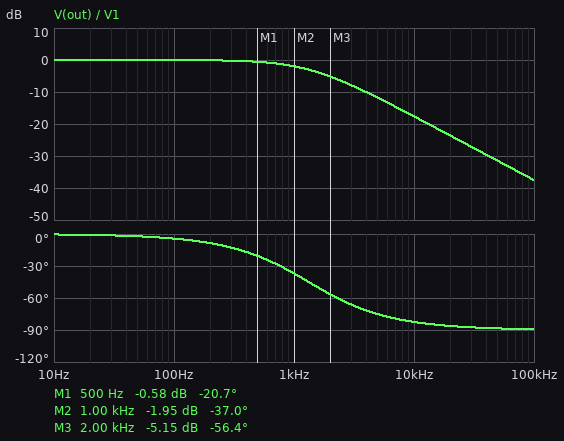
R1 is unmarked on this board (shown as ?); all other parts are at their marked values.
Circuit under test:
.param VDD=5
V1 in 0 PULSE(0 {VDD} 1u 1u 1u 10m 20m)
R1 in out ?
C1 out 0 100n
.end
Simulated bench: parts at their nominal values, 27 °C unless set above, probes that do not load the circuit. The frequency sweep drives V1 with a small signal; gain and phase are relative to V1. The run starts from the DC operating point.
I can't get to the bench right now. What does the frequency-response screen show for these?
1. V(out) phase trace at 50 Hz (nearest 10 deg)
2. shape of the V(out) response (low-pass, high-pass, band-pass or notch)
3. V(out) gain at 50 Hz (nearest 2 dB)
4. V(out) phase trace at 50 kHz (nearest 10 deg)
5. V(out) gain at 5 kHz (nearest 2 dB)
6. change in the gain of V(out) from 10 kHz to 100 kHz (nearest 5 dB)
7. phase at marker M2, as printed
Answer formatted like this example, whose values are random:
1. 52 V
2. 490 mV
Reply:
1. 0 deg
2. low-pass
3. 0 dB
4. -90 deg
5. -12 dB
6. -20 dB
7. -37.0 deg
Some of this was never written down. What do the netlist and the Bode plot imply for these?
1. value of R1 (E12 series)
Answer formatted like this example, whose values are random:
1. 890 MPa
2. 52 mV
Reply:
1. 1.2 kΩ
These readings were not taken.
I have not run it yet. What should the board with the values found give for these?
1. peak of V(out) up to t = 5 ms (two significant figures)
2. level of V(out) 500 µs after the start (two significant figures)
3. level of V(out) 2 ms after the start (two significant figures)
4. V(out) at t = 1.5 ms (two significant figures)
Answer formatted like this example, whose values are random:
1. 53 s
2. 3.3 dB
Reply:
1. 5.0 V
2. 4.9 V
3. 5.0 V
4. 5.0 V
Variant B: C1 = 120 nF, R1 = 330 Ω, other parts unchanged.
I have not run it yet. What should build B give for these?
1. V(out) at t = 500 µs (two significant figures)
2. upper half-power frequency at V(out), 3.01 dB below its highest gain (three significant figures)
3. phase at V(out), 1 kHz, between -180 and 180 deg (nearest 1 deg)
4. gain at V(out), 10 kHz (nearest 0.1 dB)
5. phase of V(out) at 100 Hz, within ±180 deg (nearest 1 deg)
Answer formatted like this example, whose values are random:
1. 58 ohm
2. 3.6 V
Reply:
1. 5.0 V
2. 4.02 kHz
3. -14 deg
4. -8.6 dB
5. -1 deg
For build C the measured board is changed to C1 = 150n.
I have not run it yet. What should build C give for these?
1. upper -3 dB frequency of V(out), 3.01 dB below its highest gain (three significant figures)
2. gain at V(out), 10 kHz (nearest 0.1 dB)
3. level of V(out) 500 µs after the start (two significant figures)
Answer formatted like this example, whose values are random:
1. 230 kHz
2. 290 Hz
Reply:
1. 884 Hz
2. -21.1 dB
3. 4.7 V
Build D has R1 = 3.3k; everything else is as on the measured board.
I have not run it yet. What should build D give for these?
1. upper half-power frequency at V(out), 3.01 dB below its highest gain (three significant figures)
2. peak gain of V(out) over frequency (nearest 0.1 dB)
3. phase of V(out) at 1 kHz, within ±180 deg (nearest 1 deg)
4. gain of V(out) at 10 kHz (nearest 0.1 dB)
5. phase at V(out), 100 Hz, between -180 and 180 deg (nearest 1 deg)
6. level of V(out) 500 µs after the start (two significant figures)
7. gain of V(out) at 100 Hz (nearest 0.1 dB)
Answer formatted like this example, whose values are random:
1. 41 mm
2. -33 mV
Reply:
1. 482 Hz
2. 0 dB
3. -64 deg
4. -26.3 dB
5. -12 deg
6. 3.9 V
7. -0.2 dB
